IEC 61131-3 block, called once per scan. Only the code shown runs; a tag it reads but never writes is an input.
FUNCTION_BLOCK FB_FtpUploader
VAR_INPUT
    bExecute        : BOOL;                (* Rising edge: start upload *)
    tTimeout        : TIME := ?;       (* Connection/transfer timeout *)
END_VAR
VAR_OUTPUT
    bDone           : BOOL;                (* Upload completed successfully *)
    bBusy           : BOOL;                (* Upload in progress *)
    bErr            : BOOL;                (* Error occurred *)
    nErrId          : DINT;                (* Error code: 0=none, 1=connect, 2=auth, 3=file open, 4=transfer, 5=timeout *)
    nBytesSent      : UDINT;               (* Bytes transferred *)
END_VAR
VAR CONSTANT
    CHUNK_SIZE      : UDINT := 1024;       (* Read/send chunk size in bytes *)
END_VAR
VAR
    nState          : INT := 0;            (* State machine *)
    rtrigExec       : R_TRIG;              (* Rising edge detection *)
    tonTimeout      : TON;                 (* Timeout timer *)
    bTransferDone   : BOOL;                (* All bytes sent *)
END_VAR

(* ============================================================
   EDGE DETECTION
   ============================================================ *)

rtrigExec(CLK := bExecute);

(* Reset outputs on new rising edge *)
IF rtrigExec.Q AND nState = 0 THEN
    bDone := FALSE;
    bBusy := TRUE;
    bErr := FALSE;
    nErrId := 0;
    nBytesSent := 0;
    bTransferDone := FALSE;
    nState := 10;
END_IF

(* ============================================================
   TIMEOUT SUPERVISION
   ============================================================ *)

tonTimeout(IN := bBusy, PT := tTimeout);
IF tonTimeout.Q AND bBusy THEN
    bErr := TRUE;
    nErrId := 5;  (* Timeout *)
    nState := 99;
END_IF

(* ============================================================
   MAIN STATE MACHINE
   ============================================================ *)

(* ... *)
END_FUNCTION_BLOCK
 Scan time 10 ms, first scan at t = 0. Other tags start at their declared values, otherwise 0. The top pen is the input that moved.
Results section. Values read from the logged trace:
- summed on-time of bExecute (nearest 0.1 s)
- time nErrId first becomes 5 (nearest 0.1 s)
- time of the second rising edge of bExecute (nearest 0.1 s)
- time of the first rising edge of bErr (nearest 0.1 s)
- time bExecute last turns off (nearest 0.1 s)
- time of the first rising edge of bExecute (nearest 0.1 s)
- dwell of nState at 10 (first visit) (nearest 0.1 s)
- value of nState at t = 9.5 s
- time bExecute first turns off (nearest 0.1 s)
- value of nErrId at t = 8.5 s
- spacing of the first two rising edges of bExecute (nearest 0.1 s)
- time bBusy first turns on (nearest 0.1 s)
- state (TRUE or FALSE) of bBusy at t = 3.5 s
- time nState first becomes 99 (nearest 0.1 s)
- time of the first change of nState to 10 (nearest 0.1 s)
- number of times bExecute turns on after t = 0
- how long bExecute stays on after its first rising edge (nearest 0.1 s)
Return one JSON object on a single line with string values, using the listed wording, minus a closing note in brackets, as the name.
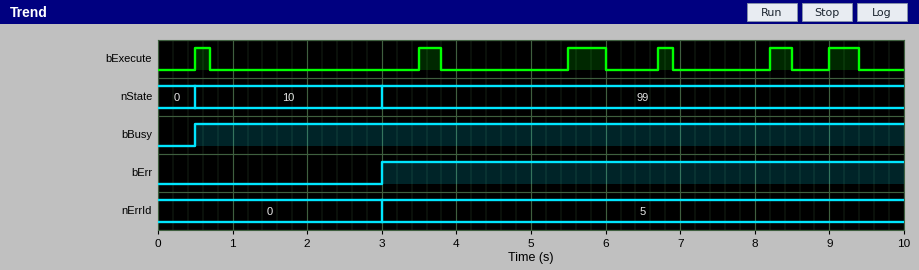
{"summed on-time of bExecute": "1.9 s", "time nErrId first becomes 5": "3.0 s", "time of the second rising edge of bExecute": "3.5 s", "time of the first rising edge of bErr": "3.0 s", "time bExecute last turns off": "9.4 s", "time of the first rising edge of bExecute": "0.5 s", "dwell of nState at 10 (first visit)": "2.5 s", "value of nState at t = 9.5 s": "99", "time bExecute first turns off": "0.7 s", "value of nErrId at t = 8.5 s": "5", "spacing of the first two rising edges of bExecute": "3.0 s", "time bBusy first turns on": "0.5 s", "state (TRUE or FALSE) of bBusy at t = 3.5 s": "TRUE", "time nState first becomes 99": "3.0 s", "time of the first change of nState to 10": "0.5 s", "number of times bExecute turns on after t = 0": "6", "how long bExecute stays on after its first rising edge": "0.2 s"}
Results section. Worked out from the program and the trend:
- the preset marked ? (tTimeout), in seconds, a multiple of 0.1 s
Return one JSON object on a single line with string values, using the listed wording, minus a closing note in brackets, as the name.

{"the preset marked ? (tTimeout), in seconds, a multiple of 0.1 s": "2.5 s"}
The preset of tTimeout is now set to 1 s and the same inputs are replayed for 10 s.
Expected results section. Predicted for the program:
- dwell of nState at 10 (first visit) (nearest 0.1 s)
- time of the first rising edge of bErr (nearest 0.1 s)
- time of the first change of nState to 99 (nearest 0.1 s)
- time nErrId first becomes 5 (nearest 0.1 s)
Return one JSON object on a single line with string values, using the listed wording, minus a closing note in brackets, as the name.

{"dwell of nState at 10 (first visit)": "1.0 s", "time of the first rising edge of bErr": "1.5 s", "time of the first change of nState to 99": "1.5 s", "time nErrId first becomes 5": "1.5 s"}
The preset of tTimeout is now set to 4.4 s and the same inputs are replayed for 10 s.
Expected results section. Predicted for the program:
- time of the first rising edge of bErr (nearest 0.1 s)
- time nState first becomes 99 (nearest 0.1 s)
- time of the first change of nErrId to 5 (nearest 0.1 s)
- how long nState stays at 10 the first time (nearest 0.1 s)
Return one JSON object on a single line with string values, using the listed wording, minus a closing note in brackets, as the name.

{"time of the first rising edge of bErr": "4.9 s", "time nState first becomes 99": "4.9 s", "time of the first change of nErrId to 5": "4.9 s", "how long nState stays at 10 the first time": "4.4 s"}
